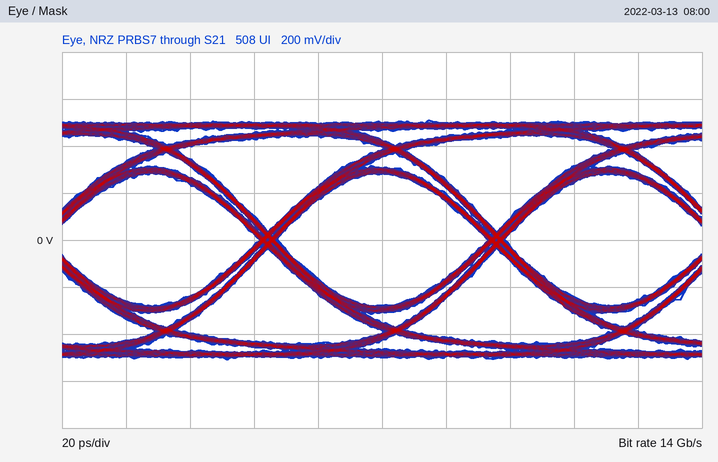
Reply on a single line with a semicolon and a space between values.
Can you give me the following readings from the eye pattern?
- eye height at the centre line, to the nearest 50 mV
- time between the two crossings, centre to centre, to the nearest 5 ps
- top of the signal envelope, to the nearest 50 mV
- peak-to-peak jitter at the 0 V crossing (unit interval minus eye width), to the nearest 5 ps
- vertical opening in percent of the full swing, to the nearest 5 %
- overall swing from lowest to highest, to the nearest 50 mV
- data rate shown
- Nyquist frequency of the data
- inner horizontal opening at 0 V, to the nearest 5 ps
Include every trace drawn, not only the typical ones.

550 mV; 70 ps; 500 mV; 5 ps; 55 %; 1.00 V; 14 Gb/s; 7 GHz; 65 ps
